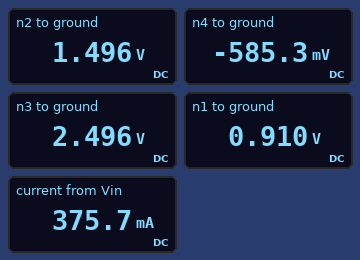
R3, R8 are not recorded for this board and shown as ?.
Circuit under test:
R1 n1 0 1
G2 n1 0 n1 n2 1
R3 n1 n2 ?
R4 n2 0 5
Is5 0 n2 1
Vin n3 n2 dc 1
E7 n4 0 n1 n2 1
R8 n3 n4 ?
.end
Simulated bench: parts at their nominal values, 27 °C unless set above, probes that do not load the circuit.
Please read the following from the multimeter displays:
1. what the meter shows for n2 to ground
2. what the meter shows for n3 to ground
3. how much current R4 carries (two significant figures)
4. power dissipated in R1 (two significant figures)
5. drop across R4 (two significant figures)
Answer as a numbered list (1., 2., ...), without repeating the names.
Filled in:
1. 1.496 V
2. 2.496 V
3. 300 mA
4. 830 mW
5. 1.5 V
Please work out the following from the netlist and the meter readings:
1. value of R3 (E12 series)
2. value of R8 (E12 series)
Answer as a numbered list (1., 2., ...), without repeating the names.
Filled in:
1. 1.8 Ω
2. 8.2 Ω
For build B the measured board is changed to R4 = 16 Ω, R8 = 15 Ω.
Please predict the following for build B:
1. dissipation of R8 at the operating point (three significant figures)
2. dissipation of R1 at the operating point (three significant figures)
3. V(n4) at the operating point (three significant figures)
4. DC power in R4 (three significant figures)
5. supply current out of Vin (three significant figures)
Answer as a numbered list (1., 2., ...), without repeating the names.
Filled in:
1. 1.34 W
2. 2.32 W
3. -980 mV
4. 392 mW
5. 299 mA
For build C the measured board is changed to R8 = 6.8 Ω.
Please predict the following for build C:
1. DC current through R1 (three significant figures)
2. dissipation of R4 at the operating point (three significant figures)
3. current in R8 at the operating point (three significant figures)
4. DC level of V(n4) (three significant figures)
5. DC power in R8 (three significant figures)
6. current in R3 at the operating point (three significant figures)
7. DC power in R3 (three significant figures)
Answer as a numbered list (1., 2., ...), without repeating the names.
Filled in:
1. 835 mA
2. 376 mW
3. 428 mA
4. -537 mV
5. 1.24 W
6. 298 mA
7. 160 mW
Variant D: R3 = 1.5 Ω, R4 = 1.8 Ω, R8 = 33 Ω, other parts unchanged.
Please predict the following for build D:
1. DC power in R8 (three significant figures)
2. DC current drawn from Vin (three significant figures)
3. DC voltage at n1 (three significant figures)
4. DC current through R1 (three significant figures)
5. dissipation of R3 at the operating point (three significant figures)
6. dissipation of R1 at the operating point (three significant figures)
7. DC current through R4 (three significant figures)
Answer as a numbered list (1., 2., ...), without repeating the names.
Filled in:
1. 201 mW
2. 78.0 mA
3. 715 mV
4. 715 mA
5. 123 mW
6. 512 mW
7. 636 mA
